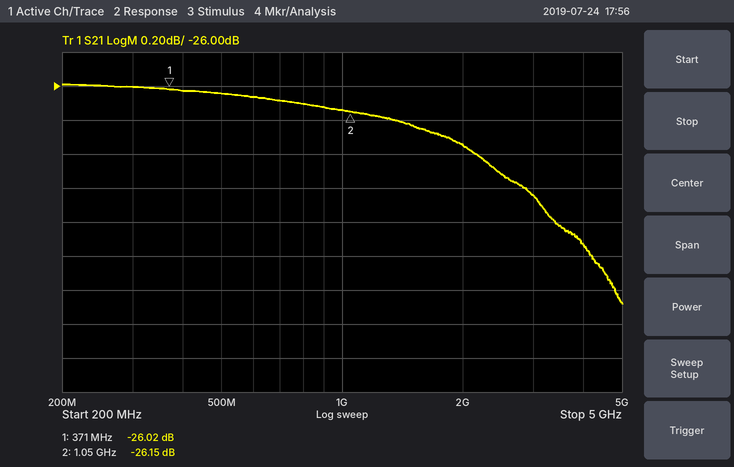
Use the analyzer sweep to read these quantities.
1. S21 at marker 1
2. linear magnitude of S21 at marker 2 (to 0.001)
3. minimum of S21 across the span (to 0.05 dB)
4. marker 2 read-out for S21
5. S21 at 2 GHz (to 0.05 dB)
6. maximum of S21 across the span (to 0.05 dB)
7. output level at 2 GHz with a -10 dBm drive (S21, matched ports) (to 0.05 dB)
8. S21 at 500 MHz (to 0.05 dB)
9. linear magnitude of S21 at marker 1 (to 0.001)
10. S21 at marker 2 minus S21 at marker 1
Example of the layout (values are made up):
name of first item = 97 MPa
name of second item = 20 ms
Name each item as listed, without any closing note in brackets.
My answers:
S21 at marker 1 = -26.02 dB
linear magnitude of S21 at marker 2 = 0.049
minimum of S21 across the span = -27.30 dB
marker 2 read-out for S21 = -26.15 dB
S21 at 2 GHz = -26.35 dB
maximum of S21 across the span = -26.00 dB
output level at 2 GHz with a -10 dBm drive (S21, matched ports) = -36.35 dBm
S21 at 500 MHz = -26.05 dB
linear magnitude of S21 at marker 1 = 0.050
S21 at marker 2 minus S21 at marker 1 = -0.13 dB
